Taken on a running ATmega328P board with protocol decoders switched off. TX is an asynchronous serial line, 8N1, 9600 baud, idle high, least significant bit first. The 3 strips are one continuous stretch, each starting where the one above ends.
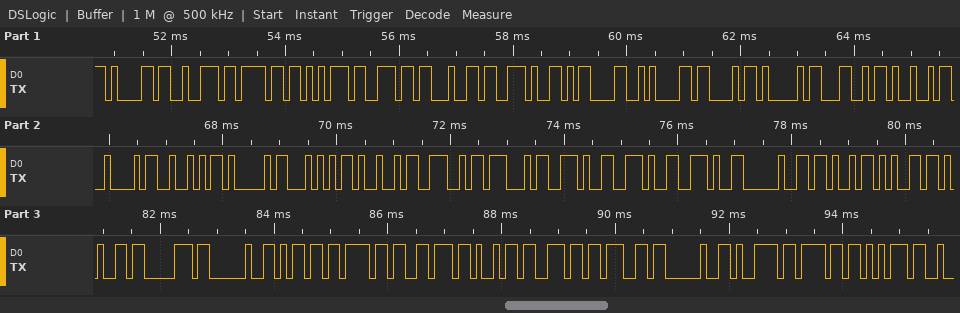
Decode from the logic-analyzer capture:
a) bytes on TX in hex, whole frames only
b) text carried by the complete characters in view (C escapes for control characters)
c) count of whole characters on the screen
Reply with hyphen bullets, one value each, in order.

- 61 72 6F 75 6E 64 2E 0D 0A 43 41 4C 49 42 52 41 54 49 4E 47 2E 2E 2E 20 4B 65 65 70 20 6D 6F 76 69 6E 67 20 79 6F 75
- "around.\r\nCALIBRATING... Keep moving you"
- 39
